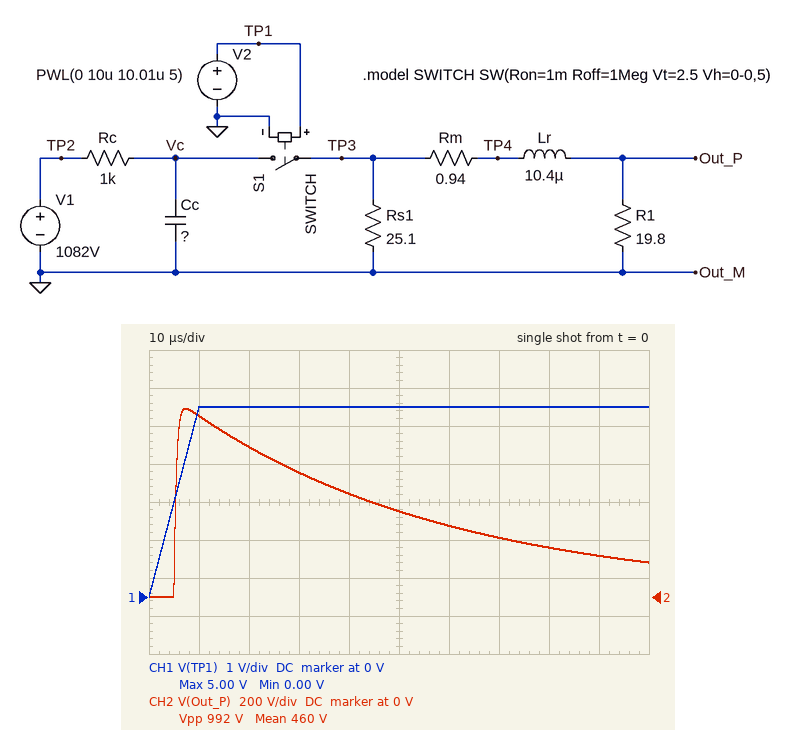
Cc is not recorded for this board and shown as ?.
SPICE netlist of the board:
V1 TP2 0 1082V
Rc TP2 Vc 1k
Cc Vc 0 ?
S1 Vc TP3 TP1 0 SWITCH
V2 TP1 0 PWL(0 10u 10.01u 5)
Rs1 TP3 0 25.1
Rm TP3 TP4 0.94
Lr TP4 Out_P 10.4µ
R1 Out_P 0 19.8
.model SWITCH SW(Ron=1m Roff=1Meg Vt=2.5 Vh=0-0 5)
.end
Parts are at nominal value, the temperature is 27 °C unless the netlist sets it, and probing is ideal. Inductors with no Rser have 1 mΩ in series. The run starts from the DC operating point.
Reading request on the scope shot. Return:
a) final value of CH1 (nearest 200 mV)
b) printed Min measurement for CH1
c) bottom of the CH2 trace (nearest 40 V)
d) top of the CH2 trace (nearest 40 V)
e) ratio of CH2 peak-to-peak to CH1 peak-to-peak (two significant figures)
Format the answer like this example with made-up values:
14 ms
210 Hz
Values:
5.0 V
0.00 V
0 V
1.00 kV
200
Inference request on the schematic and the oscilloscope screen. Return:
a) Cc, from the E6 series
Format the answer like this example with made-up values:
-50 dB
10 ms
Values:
4.7 µF
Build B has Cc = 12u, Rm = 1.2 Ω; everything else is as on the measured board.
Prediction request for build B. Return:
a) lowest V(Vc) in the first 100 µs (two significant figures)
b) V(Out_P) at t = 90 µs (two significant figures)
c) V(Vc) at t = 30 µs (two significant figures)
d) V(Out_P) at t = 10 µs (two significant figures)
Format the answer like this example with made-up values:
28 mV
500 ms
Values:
540 V
550 V
900 V
990 V
